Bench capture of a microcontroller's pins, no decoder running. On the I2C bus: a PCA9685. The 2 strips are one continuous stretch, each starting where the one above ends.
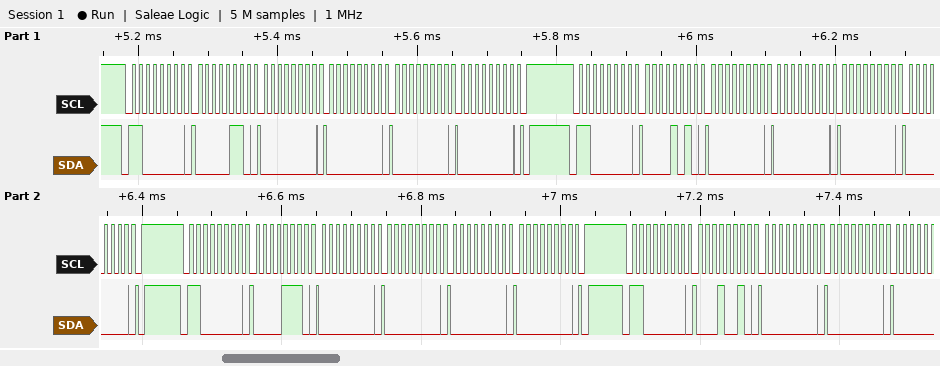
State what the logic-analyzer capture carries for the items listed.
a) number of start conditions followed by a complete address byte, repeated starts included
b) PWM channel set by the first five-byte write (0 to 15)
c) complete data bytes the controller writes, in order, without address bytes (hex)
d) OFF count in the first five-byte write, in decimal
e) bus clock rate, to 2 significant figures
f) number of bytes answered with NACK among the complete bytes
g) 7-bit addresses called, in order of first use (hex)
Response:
4
0
06 00 00 00 00 0A 00 00 00 00 0E 00 00 00 00 12 00 00
0
100 kHz
0
0x60
